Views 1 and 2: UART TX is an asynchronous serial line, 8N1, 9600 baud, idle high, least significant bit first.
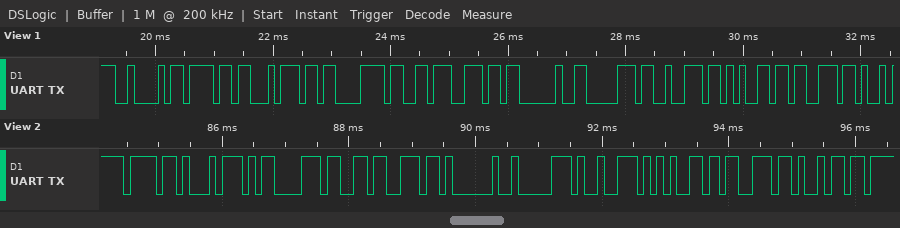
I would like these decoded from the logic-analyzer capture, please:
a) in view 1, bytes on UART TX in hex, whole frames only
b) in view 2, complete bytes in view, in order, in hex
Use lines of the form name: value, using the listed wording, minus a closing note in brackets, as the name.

in view 1, bytes on UART TX in hex, whole frames only: 0x42 0x6F 0x74 0xC3 0xB3 0x6E 0x20 0x70 0x72 0x65 0x73
in view 2, complete bytes in view, in order, in hex: 6F 74 C3 B3 6E 20 70 72 65 73 69
